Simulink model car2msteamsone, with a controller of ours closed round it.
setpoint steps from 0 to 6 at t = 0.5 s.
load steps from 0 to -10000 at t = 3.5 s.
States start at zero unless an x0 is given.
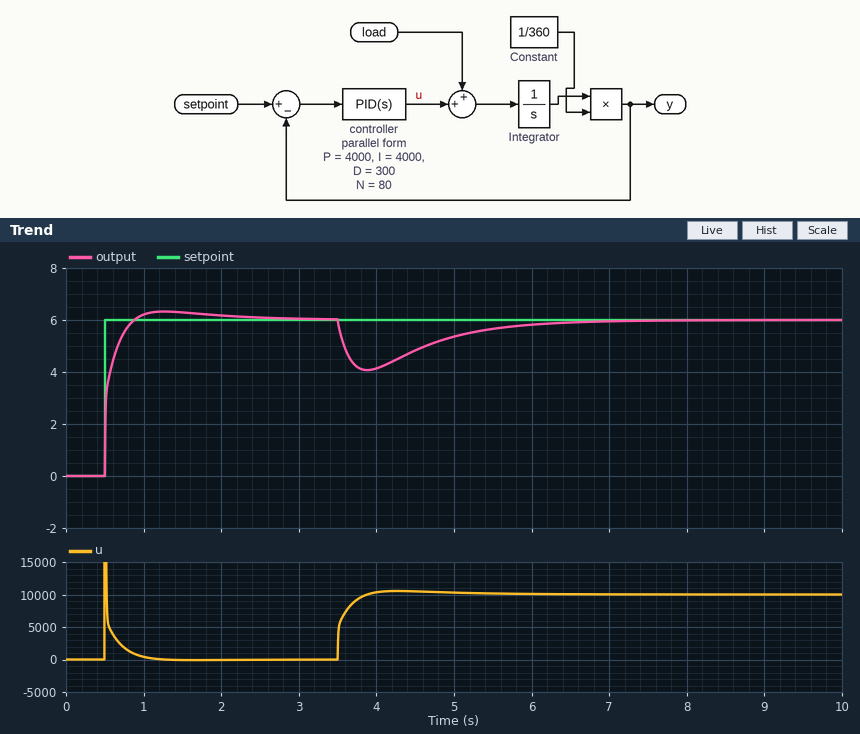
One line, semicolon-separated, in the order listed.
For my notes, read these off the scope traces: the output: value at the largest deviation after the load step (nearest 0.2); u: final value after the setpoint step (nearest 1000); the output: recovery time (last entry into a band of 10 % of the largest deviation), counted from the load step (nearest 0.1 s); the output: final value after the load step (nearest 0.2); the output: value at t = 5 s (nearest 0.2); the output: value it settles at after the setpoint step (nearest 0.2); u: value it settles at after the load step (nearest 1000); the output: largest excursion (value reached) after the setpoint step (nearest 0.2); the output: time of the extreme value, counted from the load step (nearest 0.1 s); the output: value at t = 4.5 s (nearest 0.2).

4.0; 0; 2.4 s; 6.0; 5.4; 6.0; 10000; 6.4; 0.4 s; 4.8
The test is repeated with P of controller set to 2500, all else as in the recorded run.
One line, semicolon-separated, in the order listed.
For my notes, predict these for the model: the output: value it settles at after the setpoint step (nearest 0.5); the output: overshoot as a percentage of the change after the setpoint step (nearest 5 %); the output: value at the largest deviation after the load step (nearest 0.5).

6.0; 10 %; 3.5
